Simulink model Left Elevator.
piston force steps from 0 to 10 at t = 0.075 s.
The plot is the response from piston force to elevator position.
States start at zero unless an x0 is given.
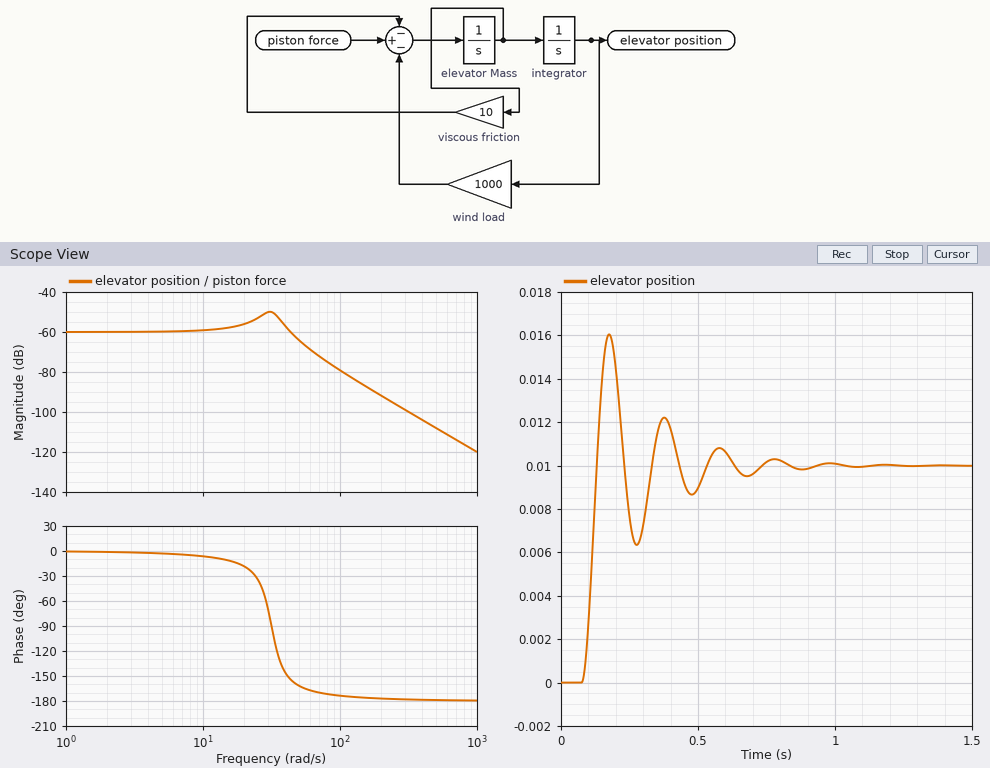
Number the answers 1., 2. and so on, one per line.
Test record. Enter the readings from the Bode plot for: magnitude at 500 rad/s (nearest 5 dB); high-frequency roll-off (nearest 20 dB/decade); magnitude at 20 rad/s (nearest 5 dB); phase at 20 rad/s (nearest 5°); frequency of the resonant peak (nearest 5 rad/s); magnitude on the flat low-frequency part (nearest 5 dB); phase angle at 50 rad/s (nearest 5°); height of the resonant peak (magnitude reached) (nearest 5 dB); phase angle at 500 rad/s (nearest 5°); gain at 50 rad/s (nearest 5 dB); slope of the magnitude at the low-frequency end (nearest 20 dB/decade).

1. -110 dB
2. -40 dB/decade
3. -55 dB
4. -20°
5. 30 rad/s
6. -60 dB
7. -160°
8. -50 dB
9. -180°
10. -65 dB
11. 0 dB/decade
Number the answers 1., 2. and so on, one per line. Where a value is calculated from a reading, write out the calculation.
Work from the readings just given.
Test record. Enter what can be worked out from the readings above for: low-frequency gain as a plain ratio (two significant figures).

1. 10^(-60 / 20) = 0.0010
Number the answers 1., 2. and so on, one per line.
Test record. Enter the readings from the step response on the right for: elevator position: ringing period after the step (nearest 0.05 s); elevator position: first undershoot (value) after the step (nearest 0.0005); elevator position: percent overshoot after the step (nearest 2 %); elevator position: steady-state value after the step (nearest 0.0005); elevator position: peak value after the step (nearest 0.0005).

1. 0.20 s
2. 0.0065
3. 60 %
4. 0.0100
5. 0.0160
